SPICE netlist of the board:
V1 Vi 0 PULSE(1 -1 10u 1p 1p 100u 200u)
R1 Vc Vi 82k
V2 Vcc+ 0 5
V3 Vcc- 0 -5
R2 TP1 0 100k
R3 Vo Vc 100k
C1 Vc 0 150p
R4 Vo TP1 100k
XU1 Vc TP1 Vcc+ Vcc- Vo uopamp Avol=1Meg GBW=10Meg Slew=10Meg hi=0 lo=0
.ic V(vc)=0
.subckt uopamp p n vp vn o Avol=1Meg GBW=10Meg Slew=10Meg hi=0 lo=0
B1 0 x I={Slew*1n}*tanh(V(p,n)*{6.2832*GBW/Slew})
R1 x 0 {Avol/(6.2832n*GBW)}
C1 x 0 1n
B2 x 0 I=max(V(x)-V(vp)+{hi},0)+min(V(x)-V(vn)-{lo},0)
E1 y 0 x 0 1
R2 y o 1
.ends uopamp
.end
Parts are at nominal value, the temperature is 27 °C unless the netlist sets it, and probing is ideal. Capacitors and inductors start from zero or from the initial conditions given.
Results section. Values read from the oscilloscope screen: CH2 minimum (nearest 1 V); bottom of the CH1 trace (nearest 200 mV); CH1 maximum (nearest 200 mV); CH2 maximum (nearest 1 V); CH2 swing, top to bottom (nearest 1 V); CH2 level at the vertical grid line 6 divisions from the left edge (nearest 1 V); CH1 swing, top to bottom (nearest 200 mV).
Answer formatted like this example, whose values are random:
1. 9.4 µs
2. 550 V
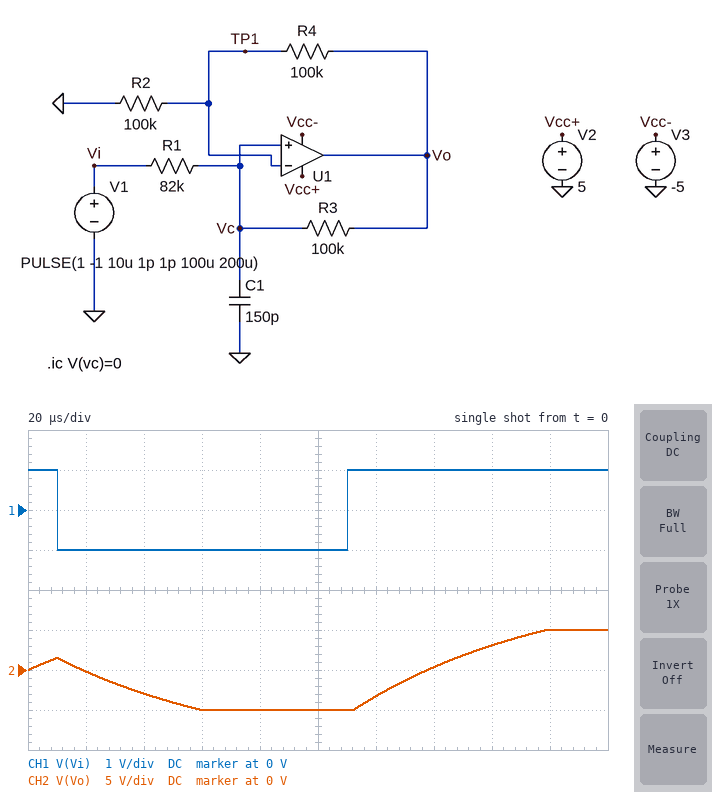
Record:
1. -5 V
2. -1.0 V
3. 1.0 V
4. 5 V
5. 10 V
6. -3 V
7. 2.0 V
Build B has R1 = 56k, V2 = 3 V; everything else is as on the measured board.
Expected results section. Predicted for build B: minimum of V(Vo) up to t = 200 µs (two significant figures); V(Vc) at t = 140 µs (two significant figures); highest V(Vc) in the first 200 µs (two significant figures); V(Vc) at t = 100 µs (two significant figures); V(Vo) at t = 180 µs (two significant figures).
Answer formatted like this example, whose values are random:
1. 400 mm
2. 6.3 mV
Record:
1. -4.5 V
2. 1.3 V
3. 1.7 V
4. -2.2 V
5. 3.0 V
